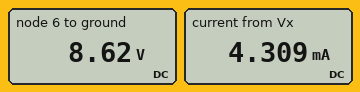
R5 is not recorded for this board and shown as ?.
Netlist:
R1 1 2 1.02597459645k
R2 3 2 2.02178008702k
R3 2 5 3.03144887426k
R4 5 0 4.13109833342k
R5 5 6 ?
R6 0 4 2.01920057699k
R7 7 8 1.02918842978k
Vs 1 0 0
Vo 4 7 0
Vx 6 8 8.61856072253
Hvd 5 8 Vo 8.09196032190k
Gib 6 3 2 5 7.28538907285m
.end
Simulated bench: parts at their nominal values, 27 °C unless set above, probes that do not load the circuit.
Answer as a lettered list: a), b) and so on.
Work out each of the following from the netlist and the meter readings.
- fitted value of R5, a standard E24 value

a) 2 kΩ
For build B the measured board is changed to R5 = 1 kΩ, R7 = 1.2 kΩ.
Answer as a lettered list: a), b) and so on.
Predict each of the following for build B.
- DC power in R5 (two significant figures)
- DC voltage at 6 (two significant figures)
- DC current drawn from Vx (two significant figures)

a) 74 mW
b) 8.6 V
c) 8.6 mA
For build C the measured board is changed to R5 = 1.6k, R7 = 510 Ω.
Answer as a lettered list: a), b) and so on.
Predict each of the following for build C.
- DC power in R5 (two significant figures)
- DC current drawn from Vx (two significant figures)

a) 46 mW
b) 5.4 mA
